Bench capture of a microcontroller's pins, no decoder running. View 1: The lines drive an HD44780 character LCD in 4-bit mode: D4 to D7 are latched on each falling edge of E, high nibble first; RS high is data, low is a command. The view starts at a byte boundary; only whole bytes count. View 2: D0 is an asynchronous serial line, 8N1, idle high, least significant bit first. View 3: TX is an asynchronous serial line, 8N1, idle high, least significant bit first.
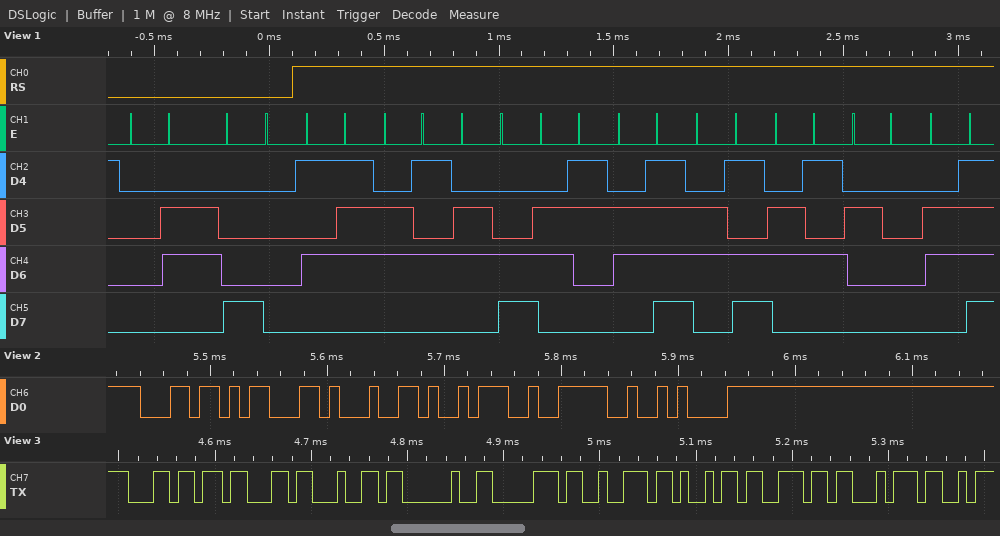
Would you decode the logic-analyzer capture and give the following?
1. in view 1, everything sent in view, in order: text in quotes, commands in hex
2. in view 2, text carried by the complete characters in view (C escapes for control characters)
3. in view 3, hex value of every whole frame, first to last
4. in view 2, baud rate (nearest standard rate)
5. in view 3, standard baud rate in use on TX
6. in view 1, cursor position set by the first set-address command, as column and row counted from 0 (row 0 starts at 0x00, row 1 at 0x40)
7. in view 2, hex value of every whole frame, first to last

0x06 0x80 "Welcome o"
"lcd:>\n"
6C 63 64 20 70 72 69 6E 74
115200 baud
115200 baud
column 0, row 0
6C 63 64 3A 3E 0A
